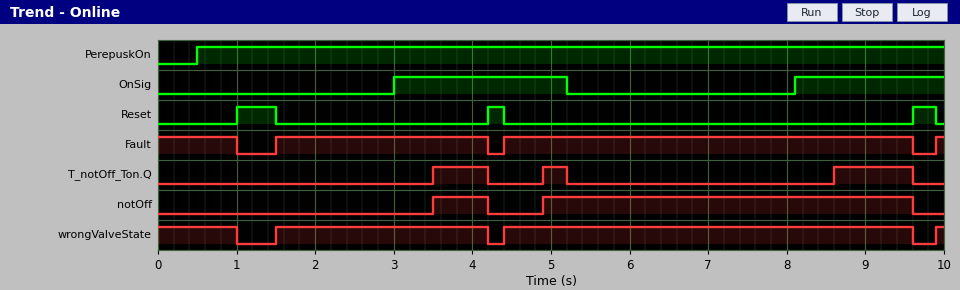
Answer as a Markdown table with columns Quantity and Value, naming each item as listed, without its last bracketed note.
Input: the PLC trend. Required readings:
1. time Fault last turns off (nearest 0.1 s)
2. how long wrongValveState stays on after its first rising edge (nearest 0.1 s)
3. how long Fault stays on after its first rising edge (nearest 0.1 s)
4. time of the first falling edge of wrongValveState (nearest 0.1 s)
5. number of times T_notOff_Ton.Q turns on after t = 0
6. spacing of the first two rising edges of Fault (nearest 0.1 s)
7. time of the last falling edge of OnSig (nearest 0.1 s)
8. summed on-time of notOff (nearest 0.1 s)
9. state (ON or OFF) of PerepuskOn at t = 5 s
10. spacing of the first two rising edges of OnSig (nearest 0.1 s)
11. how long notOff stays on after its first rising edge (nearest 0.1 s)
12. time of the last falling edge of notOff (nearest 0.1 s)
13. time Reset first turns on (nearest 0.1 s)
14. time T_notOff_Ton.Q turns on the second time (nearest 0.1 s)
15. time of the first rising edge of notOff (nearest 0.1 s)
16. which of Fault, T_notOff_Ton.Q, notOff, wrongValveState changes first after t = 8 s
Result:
| Quantity | Value |
|---|---|
| time Fault last turns off | 9.6 s |
| how long wrongValveState stays on after its first rising edge | 2.7 s |
| how long Fault stays on after its first rising edge | 2.7 s |
| time of the first falling edge of wrongValveState | 1.0 s |
| number of times T_notOff_Ton.Q turns on after t = 0 | 3 |
| spacing of the first two rising edges of Fault | 2.9 s |
| time of the last falling edge of OnSig | 5.2 s |
| summed on-time of notOff | 5.4 s |
| state (ON or OFF) of PerepuskOn at t = 5 s | ON |
| spacing of the first two rising edges of OnSig | 5.1 s |
| how long notOff stays on after its first rising edge | 0.7 s |
| time of the last falling edge of notOff | 9.6 s |
| time Reset first turns on | 1.0 s |
| time T_notOff_Ton.Q turns on the second time | 4.9 s |
| time of the first rising edge of notOff | 3.5 s |
| which of Fault, T_notOff_Ton.Q, notOff, wrongValveState changes first after t = 8 s | T_notOff_Ton.Q |
